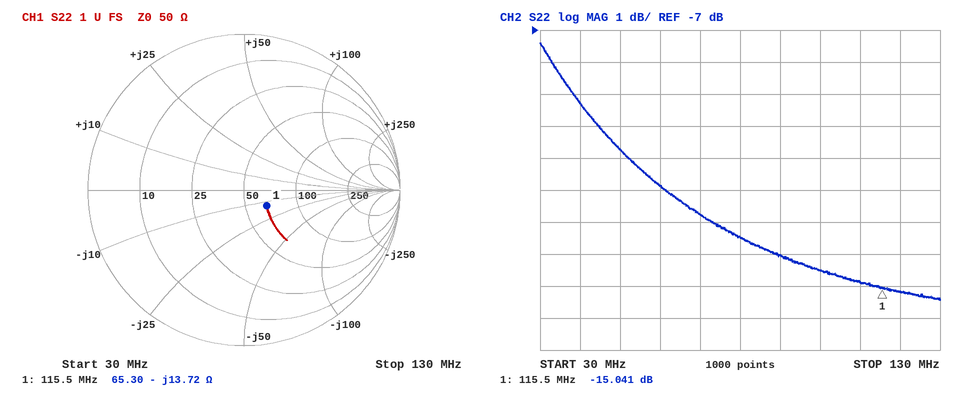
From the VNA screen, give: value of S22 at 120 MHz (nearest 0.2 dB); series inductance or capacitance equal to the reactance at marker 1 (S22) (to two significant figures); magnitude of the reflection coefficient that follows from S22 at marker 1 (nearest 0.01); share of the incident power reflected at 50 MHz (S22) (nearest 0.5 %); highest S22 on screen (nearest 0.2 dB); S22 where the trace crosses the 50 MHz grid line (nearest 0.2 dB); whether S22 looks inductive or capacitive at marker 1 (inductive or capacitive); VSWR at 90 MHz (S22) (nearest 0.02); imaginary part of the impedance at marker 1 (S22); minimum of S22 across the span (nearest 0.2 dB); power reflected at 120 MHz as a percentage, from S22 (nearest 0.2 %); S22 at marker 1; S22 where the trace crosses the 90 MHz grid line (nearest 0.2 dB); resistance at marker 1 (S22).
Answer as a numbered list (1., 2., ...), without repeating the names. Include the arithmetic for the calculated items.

1. -15.2 dB
2. C = 1/(2π × 115.5 MHz × 13.72 Ω) ≈ 100 pF
3. 10^(-15.041/20) ≈ 0.18
4. 10^(-10.8/10) ≈ 8.32 %, so 8.5 % to the nearest 0.5 %
5. -7.4 dB
6. -10.8 dB
7. capacitive
8. |Γ| = 10^(-14/20) = 0.1995; VSWR = (1 + 0.1995)/(1 − 0.1995) ≈ 1.50
9. -13.72 Ω
10. -15.4 dB
11. 10^(-15.2/10) ≈ 3.0 %
12. -15.041 dB
13. -14.0 dB
14. 65.30 Ω
